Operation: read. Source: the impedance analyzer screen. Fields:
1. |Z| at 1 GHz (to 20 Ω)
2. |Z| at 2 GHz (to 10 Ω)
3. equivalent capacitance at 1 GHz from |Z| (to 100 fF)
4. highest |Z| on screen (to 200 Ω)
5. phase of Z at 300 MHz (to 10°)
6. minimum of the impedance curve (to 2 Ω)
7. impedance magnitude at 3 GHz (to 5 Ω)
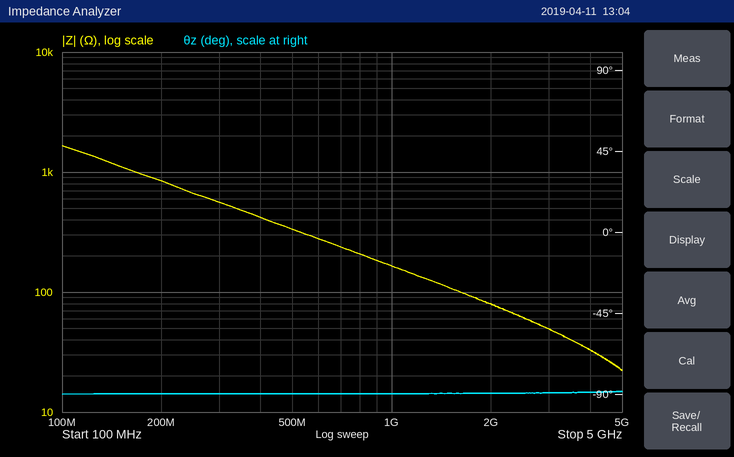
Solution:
160 Ω
80 Ω
1.0 pF
1.6 kΩ
-90°
22 Ω
50 Ω
